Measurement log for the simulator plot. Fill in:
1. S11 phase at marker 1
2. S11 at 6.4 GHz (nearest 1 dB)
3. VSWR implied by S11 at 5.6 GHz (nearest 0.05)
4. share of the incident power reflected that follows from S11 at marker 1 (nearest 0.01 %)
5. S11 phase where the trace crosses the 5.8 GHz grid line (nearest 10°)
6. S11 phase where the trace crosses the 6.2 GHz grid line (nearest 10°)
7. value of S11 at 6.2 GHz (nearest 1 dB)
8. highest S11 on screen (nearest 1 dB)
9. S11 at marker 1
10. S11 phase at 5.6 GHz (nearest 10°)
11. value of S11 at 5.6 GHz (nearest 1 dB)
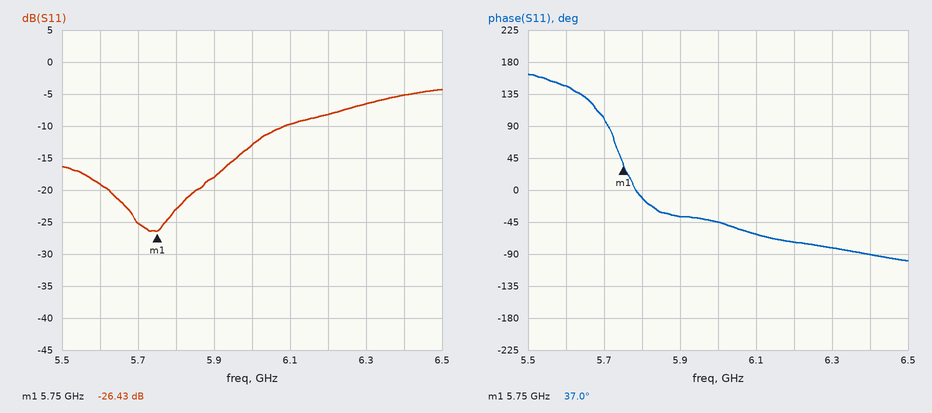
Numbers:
37.0°
-5 dB
1.25
0.23 %
-10°
-70°
-8 dB
-4 dB
-26.43 dB
150°
-19 dB
